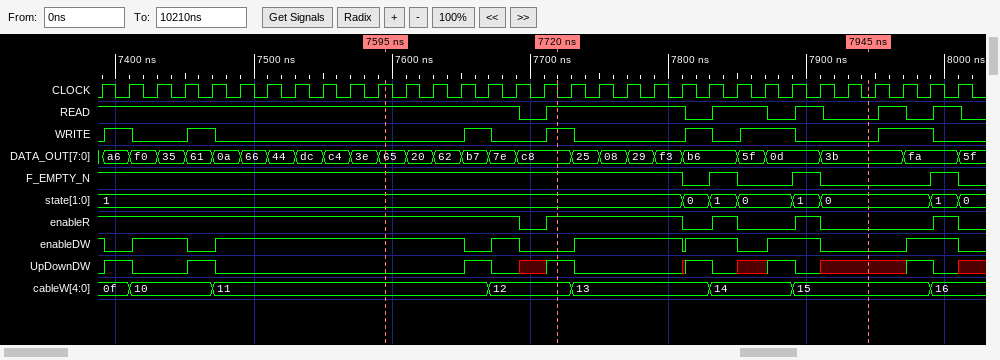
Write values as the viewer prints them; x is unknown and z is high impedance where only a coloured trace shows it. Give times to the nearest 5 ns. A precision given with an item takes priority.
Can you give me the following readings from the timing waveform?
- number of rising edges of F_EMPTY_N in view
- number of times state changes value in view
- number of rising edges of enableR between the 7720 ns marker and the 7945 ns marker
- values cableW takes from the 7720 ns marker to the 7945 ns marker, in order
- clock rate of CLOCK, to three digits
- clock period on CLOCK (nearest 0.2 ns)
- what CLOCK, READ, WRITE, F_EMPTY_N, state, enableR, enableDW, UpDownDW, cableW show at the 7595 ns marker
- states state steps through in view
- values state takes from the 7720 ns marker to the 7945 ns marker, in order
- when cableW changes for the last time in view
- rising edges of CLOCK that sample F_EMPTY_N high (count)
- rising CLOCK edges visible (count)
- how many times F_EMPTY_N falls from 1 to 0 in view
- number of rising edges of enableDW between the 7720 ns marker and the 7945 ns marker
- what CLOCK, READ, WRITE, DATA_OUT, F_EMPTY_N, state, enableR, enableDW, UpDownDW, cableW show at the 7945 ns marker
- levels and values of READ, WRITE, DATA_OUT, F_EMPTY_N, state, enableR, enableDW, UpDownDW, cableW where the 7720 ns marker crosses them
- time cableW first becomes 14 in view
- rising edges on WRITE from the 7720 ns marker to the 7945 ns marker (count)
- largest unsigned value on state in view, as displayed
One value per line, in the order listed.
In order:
3
7
2
12, 13, 14, 15
50.0 MHz
20 ns
CLOCK=1, READ=1, WRITE=0, F_EMPTY_N=1, state=1, enableR=1, enableDW=1, UpDownDW=0, cableW=11
1, 0, 1, 0, 1, 0, 1, 0
1, 0, 1, 0, 1, 0
7990 ns
25
32
4
3
CLOCK=0, READ=0, WRITE=0, DATA_OUT=3b, F_EMPTY_N=0, state=0, enableR=0, enableDW=0, UpDownDW=x, cableW=15
READ=1, WRITE=1, DATA_OUT=c8, F_EMPTY_N=1, state=1, enableR=1, enableDW=0, UpDownDW=1, cableW=12
7830 ns
2
1
